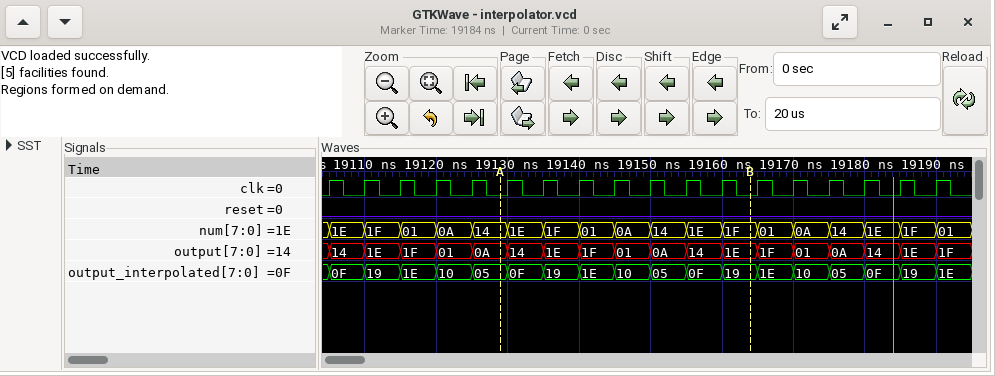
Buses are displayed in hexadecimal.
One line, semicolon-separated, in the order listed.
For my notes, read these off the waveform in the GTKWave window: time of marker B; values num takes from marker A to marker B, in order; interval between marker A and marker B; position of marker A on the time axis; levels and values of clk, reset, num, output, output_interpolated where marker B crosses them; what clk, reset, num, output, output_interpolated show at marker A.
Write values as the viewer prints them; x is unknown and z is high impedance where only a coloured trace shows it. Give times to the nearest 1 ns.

19164 ns; 14, 1E, 1F, 01, 0A, 14, 1E, 1F; 35 ns; 19129 ns; clk=0, reset=0, num=1F, output=1E, output_interpolated=19; clk=0, reset=0, num=14, output=0A, output_interpolated=05
